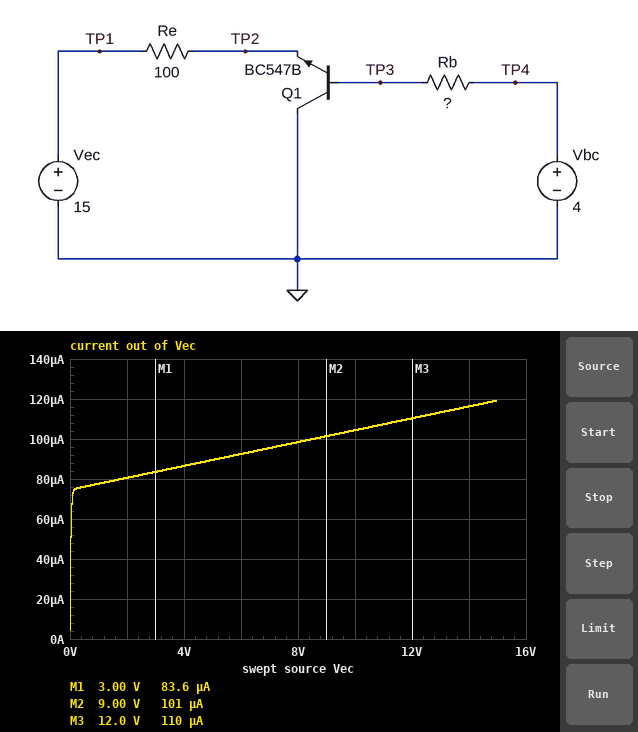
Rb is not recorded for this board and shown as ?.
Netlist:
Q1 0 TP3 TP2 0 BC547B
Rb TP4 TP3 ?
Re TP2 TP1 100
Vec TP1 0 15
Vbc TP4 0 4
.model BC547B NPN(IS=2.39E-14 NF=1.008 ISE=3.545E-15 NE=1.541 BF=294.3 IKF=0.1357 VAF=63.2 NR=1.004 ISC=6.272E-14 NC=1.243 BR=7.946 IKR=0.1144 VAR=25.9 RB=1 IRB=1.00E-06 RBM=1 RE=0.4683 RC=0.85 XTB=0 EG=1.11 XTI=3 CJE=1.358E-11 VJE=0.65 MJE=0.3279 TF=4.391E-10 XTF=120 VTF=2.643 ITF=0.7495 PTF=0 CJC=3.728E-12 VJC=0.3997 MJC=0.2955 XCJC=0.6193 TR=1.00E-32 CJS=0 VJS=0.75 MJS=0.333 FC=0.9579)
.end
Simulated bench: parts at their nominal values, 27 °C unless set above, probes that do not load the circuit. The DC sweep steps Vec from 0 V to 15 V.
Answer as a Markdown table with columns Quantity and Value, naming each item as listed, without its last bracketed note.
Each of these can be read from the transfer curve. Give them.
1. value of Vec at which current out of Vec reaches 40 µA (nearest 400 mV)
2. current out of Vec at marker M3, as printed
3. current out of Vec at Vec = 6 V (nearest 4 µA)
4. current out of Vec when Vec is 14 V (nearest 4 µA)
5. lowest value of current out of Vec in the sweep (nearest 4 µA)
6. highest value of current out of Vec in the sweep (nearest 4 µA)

| Quantity | Value |
|---|---|
| value of Vec at which current out of Vec reaches 40 µA | 0 V |
| current out of Vec at marker M3, as printed | 110 µA |
| current out of Vec at Vec = 6 V | 92 µA |
| current out of Vec when Vec is 14 V | 116 µA |
| lowest value of current out of Vec in the sweep | 4 µA |
| highest value of current out of Vec in the sweep | 120 µA |
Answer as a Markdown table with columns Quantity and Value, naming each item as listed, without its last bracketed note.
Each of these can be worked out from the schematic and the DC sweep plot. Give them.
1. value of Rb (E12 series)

| Quantity | Value |
|---|---|
| value of Rb | 270 kΩ |
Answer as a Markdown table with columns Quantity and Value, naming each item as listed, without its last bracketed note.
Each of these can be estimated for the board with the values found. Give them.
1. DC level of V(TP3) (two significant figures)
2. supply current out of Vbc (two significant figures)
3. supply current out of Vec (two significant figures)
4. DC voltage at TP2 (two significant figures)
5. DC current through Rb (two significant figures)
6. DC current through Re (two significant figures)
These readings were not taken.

| Quantity | Value |
|---|---|
| DC level of V(TP3) | 570 mV |
| supply current out of Vbc | 13 µA |
| supply current out of Vec | 120 µA |
| DC voltage at TP2 | 15 V |
| DC current through Rb | 13 µA |
| DC current through Re | 120 µA |
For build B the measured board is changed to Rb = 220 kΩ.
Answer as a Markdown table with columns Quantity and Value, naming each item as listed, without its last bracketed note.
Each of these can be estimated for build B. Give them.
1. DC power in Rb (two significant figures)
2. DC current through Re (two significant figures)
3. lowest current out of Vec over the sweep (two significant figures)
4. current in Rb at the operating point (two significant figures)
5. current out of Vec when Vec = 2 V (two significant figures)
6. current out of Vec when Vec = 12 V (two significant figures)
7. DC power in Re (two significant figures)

| Quantity | Value |
|---|---|
| DC power in Rb | 53 µW |
| DC current through Re | 150 µA |
| lowest current out of Vec over the sweep | 5.5 µA |
| current in Rb at the operating point | 16 µA |
| current out of Vec when Vec = 2 V | 100 µA |
| current out of Vec when Vec = 12 V | 140 µA |
| DC power in Re | 2.2 µW |
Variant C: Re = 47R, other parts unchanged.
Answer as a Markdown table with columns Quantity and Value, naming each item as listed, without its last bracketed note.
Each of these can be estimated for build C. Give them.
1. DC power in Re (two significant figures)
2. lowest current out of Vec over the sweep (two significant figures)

| Quantity | Value |
|---|---|
| DC power in Re | 670 nW |
| lowest current out of Vec over the sweep | 5.2 µA |
